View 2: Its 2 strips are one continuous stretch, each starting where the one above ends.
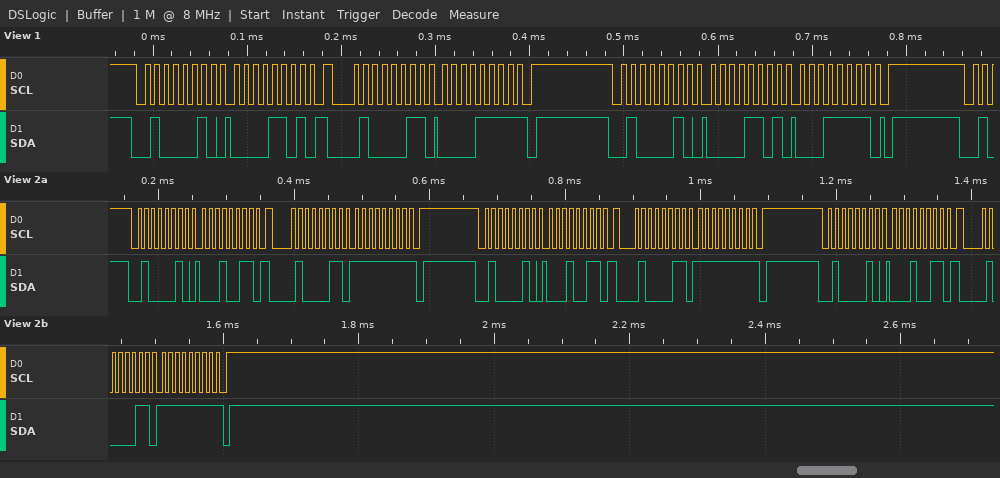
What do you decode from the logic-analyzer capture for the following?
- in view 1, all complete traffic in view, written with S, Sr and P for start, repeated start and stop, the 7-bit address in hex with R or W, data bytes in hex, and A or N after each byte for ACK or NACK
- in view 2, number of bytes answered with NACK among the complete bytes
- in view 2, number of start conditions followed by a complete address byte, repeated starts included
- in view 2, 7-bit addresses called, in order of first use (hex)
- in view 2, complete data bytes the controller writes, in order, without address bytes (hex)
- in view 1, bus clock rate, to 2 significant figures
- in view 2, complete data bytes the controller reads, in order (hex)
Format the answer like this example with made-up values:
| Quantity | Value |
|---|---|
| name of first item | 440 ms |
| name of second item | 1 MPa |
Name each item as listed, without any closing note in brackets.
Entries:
| Quantity | Value |
|---|---|
| in view 1, all complete traffic in view, written with S, Sr and P for start, repeated start and stop, the 7-bit address in hex with R or W, data bytes in hex, and A or N after each byte for ACK or NACK | S 21W A 0D A Sr 21R A 0F N P S 21W A 0D A 1F A P |
| in view 2, number of bytes answered with NACK among the complete bytes | 3 |
| in view 2, number of start conditions followed by a complete address byte, repeated starts included | 6 |
| in view 2, 7-bit addresses called, in order of first use | 0x21 |
| in view 2, complete data bytes the controller writes, in order, without address bytes | 13 13 13 |
| in view 1, bus clock rate, to 2 significant figures | 100 kHz |
| in view 2, complete data bytes the controller reads, in order | FF FF FF |
